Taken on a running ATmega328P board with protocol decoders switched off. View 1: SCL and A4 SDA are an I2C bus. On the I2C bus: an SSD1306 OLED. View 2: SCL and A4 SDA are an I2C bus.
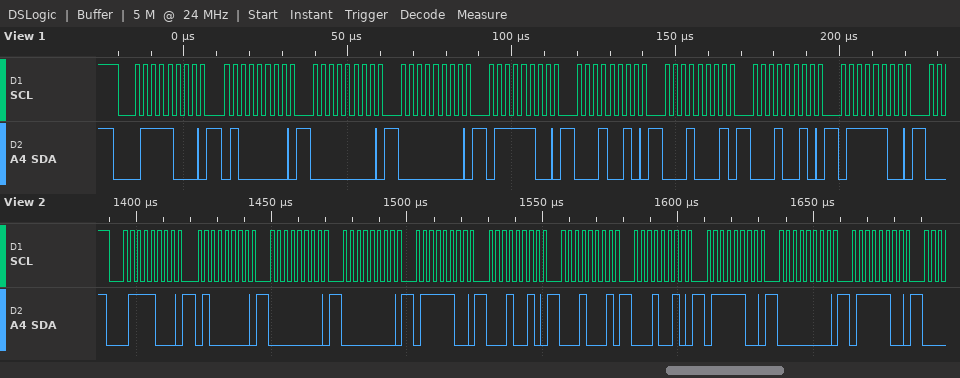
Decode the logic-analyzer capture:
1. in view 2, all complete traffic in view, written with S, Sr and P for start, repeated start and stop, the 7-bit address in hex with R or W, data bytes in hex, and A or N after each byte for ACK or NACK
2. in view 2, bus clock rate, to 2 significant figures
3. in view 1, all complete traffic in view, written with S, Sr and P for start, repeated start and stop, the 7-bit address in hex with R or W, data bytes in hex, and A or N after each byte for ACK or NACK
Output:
S 3CW A 40 A 00 A 00 A 7C A 12 A 11 A 12 A 7C A 00 A 7C A
400 kHz
S 3CW A 40 A 00 A 00 A 7C A 12 A 11 A 12 A 7C A
